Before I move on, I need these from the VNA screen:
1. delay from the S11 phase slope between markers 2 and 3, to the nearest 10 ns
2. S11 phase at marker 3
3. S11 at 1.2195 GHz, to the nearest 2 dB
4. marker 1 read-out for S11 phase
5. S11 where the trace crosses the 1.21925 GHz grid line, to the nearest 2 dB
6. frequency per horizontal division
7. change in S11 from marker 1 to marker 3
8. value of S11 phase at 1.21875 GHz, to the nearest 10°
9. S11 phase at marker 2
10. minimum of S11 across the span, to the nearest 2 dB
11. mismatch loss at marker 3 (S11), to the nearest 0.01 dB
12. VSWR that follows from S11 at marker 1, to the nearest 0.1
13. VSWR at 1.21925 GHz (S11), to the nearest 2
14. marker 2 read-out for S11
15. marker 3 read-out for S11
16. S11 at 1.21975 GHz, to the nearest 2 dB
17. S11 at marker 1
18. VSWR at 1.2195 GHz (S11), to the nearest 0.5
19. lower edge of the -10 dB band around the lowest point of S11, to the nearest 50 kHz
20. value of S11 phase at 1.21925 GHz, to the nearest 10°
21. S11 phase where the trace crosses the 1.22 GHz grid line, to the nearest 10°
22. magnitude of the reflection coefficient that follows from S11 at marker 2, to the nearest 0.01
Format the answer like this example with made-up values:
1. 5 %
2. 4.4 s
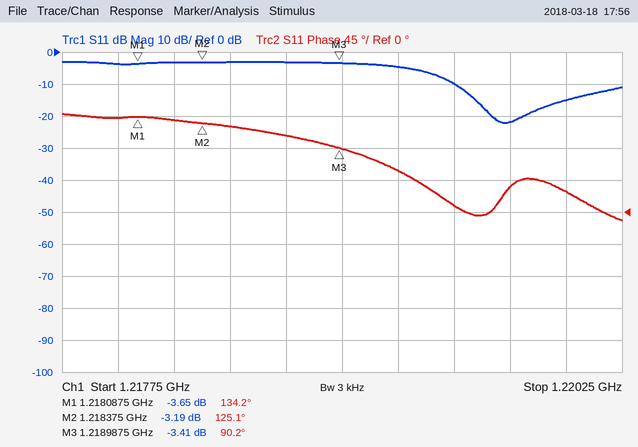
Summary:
1. 160 ns
2. 90.2°
3. -10 dB
4. 134.2°
5. -4 dB
6. 250 kHz
7. 0.24 dB
8. 110°
9. 125.1°
10. -22 dB
11. 2.64 dB
12. 4.8
13. 4
14. -3.19 dB
15. -3.41 dB
16. -22 dB
17. -3.65 dB
18. 2.0
19. 1.21950 GHz
20. 60°
21. 30°
22. 0.69
